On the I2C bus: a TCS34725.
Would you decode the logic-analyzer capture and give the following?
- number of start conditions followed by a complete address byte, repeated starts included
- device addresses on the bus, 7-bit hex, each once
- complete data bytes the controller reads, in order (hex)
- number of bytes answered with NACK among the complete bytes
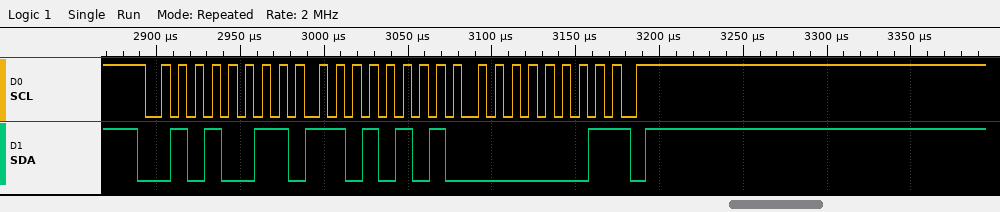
1
0x29
D5 01
1
